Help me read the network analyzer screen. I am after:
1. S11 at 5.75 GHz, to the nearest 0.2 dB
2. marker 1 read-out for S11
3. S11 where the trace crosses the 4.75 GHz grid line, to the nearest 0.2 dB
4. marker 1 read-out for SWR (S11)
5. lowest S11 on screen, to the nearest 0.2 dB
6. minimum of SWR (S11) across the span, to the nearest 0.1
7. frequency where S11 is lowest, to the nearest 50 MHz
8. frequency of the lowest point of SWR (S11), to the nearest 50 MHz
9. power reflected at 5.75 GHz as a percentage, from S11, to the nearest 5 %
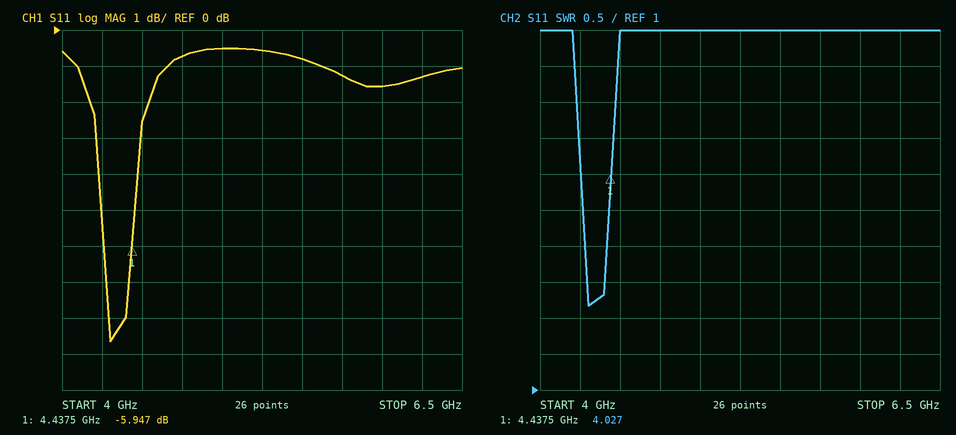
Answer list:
-1.2 dB
-5.947 dB
-0.8 dB
4.027
-8.6 dB
2.2
4.30 GHz
4.30 GHz
75 %
